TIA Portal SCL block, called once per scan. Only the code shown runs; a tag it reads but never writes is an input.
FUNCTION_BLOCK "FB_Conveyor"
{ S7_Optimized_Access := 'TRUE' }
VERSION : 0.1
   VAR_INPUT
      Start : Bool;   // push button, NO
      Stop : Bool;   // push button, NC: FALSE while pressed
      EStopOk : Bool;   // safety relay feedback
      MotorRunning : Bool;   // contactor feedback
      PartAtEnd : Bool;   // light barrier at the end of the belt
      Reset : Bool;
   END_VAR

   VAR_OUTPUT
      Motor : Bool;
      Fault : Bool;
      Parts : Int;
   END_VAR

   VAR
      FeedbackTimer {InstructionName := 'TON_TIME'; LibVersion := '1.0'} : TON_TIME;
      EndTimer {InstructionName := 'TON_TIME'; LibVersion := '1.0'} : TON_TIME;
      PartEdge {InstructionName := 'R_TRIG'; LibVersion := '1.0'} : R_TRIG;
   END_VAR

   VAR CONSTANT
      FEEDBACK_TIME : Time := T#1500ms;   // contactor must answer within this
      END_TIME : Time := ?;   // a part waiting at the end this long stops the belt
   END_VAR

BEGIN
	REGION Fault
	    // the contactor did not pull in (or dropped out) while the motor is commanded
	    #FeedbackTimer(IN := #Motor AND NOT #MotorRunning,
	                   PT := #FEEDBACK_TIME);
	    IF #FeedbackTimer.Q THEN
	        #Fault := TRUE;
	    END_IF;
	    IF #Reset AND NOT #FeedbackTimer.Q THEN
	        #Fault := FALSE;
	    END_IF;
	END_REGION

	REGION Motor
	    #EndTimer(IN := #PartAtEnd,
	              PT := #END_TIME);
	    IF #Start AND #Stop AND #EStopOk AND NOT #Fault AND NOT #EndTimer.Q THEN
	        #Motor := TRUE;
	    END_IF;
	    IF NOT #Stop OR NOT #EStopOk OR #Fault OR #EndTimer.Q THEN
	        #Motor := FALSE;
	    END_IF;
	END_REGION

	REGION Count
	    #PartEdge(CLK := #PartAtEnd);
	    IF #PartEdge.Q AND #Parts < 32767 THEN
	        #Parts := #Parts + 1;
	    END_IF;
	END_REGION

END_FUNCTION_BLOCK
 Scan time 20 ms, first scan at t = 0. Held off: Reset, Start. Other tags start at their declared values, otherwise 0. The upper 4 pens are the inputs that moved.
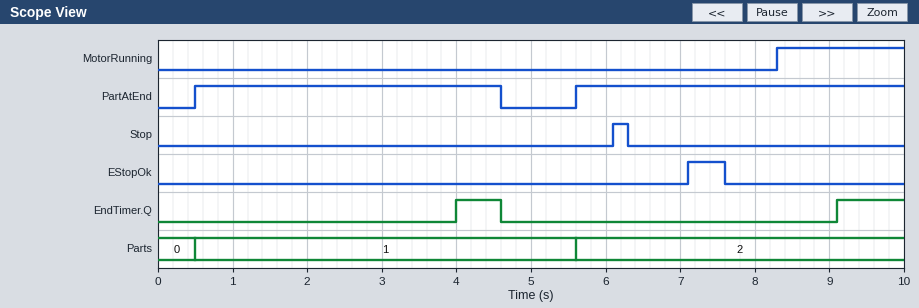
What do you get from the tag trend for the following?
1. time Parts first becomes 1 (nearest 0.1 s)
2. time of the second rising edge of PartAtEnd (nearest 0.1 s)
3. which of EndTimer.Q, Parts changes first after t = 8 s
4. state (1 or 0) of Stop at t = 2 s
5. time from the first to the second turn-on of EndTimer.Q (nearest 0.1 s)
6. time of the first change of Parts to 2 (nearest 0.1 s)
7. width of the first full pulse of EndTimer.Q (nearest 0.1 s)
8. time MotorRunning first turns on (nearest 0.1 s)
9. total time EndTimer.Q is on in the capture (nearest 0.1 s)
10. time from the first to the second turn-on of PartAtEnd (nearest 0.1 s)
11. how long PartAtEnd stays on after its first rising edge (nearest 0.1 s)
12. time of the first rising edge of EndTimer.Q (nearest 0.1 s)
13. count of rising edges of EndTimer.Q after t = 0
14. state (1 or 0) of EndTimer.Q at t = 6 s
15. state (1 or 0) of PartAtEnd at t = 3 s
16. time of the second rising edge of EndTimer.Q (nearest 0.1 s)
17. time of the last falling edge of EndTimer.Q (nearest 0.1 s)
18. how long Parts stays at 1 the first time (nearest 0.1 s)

0.5 s
5.6 s
EndTimer.Q
0
5.1 s
5.6 s
0.6 s
8.3 s
1.5 s
5.1 s
4.1 s
4.0 s
2
0
1
9.1 s
4.6 s
5.1 s
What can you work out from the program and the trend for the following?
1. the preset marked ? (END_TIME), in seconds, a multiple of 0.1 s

3.5 s
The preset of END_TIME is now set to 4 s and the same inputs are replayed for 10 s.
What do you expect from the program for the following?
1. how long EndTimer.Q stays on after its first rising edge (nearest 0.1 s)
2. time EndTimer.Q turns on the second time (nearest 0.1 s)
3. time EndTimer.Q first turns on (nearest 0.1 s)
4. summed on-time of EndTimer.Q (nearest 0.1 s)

0.1 s
9.6 s
4.5 s
0.5 s
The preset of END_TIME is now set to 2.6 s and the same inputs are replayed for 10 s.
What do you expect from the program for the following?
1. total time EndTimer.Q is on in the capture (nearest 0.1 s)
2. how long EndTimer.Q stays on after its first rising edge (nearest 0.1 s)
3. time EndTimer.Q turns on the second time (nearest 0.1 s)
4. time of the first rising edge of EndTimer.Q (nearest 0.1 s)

3.3 s
1.5 s
8.2 s
3.1 s
